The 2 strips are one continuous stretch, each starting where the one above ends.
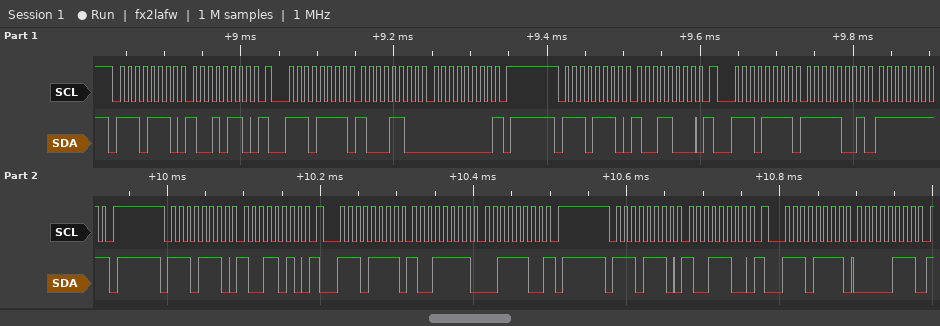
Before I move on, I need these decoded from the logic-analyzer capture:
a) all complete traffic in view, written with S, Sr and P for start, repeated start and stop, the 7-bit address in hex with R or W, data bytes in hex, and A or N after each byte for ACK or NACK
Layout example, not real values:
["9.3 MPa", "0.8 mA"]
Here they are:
["S 77W A 96 A Sr 77R A 8C A 00 N P S 77W A 98 A Sr 77R A F9 A FF N P S 77W A 9A A Sr 77R A 9F A 3C N P S 77W A 9C A Sr 77R A 07 A"]
